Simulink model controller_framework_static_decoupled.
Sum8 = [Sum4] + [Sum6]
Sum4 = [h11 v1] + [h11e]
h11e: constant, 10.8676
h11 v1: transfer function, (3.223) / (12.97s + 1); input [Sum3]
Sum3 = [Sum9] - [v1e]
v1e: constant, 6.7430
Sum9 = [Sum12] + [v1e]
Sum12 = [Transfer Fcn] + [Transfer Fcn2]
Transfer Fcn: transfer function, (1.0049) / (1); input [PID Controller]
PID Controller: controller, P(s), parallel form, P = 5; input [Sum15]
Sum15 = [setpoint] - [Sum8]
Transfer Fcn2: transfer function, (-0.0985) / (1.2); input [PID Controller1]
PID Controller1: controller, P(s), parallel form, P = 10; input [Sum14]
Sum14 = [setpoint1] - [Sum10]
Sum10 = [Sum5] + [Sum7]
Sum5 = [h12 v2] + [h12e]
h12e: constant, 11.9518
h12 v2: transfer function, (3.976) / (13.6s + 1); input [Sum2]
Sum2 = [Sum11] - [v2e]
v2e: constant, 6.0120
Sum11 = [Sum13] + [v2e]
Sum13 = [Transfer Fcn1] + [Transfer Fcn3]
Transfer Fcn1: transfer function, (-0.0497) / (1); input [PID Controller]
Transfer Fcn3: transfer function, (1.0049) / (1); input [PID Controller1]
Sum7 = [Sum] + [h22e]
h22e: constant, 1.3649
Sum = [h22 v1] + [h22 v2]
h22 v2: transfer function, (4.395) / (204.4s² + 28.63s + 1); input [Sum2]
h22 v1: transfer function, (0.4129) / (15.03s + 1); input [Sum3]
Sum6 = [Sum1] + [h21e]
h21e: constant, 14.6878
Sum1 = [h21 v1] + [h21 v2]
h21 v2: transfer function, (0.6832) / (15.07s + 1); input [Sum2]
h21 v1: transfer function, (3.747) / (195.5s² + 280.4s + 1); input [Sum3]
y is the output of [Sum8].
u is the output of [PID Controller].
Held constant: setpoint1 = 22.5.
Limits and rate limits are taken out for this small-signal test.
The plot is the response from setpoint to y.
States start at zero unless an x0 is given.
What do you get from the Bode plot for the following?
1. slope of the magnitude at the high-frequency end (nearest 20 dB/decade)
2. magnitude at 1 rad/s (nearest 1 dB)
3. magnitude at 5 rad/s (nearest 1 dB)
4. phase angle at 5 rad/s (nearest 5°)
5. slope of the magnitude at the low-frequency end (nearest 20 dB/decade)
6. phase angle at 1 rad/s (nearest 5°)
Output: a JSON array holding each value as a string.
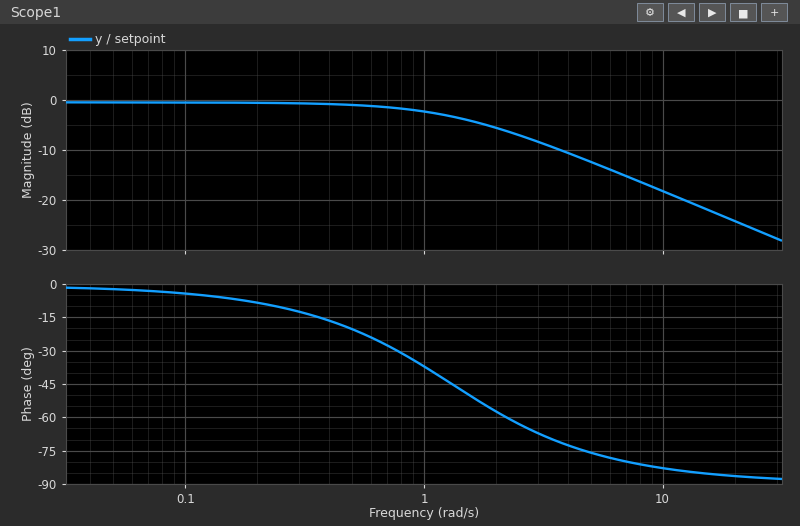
["-20 dB/decade", "-2 dB", "-12 dB", "-75°", "0 dB/decade", "-35°"]
